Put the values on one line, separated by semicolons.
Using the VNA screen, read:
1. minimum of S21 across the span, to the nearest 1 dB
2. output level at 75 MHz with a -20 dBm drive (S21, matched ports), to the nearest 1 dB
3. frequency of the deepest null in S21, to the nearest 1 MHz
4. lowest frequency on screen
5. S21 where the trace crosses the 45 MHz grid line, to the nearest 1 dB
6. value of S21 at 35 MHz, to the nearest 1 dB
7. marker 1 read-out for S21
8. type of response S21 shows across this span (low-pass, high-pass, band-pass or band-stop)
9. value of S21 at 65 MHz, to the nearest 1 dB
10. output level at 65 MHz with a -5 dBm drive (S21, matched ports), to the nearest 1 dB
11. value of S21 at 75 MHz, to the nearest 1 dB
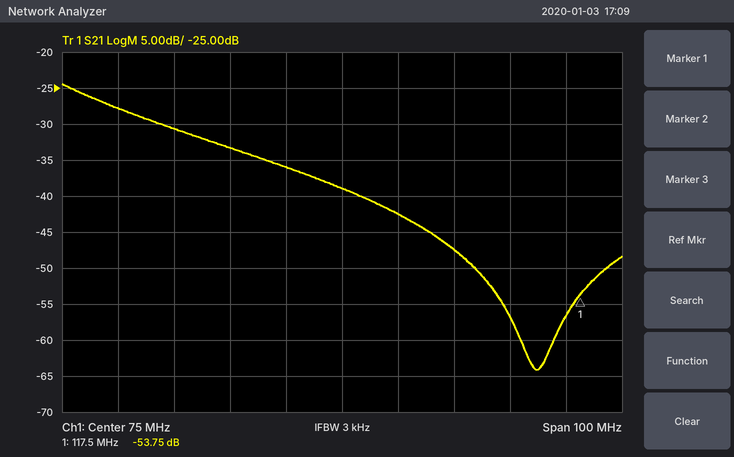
-64 dB; -59 dBm; 110 MHz; 25 MHz; -31 dB; -28 dB; -53.75 dB; low-pass; -36 dB; -41 dBm; -39 dB
